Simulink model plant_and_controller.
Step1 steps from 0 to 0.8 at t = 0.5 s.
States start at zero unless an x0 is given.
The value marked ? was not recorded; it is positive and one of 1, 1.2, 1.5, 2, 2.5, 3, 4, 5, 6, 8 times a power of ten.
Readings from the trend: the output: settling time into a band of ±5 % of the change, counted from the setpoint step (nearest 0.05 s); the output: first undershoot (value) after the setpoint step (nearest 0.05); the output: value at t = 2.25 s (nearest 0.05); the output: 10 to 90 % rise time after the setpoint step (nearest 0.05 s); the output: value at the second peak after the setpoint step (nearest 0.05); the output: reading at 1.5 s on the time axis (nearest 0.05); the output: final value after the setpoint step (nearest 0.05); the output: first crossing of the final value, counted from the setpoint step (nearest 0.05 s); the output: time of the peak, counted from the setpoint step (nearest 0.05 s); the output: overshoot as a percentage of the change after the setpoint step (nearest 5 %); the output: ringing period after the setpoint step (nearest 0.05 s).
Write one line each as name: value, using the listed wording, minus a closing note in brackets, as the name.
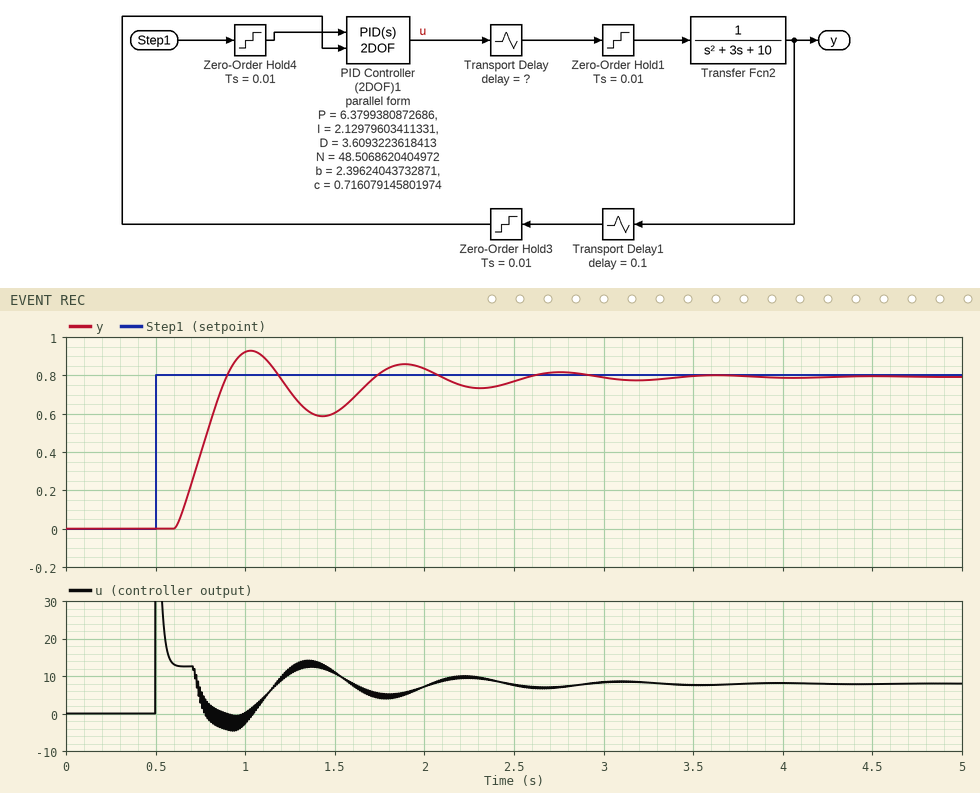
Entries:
the output: settling time into a band of ±5 % of the change, counted from the setpoint step: 1.95 s
the output: first undershoot (value) after the setpoint step: 0.60
the output: value at t = 2.25 s: 0.75
the output: 10 to 90 % rise time after the setpoint step: 0.20 s
the output: value at the second peak after the setpoint step: 0.85
the output: reading at 1.5 s on the time axis: 0.60
the output: final value after the setpoint step: 0.80
the output: first crossing of the final value, counted from the setpoint step: 0.40 s
the output: time of the peak, counted from the setpoint step: 0.55 s
the output: overshoot as a percentage of the change after the setpoint step: 15 %
the output: ringing period after the setpoint step: 0.85 s
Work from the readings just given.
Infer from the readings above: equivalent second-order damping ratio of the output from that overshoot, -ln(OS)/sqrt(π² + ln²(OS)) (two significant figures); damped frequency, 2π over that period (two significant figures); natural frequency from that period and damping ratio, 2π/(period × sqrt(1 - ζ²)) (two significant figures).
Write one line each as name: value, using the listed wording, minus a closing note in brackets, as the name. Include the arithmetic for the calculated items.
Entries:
equivalent second-order damping ratio of the output from that overshoot, -ln(OS)/sqrt(π² + ln²(OS)): ln(0.15) = -1.897; 1.897 / sqrt(9.870 + 3.599) = 0.52
damped frequency, 2π over that period: 2π / 0.85 = 7.4 rad/s
natural frequency from that period and damping ratio, 2π/(period × sqrt(1 - ζ²)): 2π / (0.85 × sqrt(1 - 0.52²)) = 8.7 rad/s
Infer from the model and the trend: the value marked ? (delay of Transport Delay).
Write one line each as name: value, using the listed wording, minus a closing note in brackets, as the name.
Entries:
the value marked ?: 0.1
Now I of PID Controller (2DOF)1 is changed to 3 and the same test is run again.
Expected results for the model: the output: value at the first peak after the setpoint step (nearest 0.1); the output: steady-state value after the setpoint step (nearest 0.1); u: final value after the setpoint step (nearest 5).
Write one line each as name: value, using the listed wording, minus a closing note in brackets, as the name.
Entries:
the output: value at the first peak after the setpoint step: 0.9
the output: steady-state value after the setpoint step: 0.8
u: final value after the setpoint step: 10
